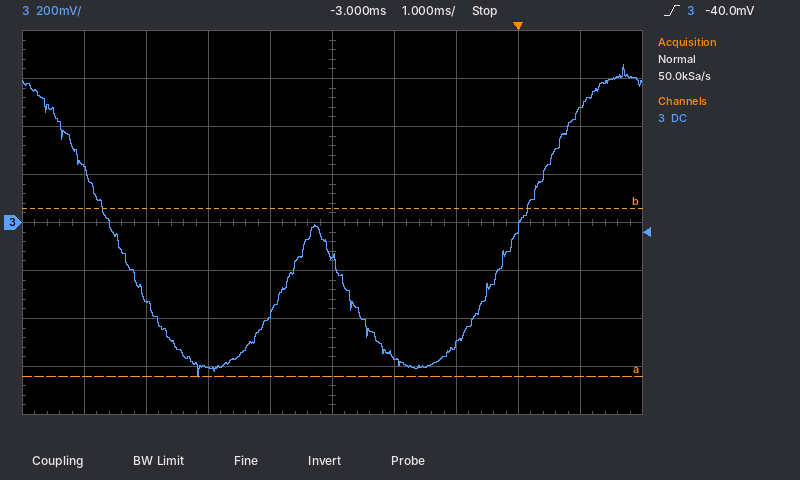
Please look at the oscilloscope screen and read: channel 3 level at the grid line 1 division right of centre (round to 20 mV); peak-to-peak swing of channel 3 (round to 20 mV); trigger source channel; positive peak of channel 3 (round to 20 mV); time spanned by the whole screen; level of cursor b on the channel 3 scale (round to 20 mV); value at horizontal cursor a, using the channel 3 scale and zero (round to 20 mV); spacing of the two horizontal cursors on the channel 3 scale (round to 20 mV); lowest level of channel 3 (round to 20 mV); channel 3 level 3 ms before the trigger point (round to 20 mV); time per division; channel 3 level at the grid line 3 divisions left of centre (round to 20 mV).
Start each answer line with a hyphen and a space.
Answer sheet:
- -560 mV
- 1.30 V
- channel 3
- 660 mV
- 10 ms
- 60 mV
- -640 mV
- 700 mV
- -640 mV
- -140 mV
- 1 ms
- -320 mV
